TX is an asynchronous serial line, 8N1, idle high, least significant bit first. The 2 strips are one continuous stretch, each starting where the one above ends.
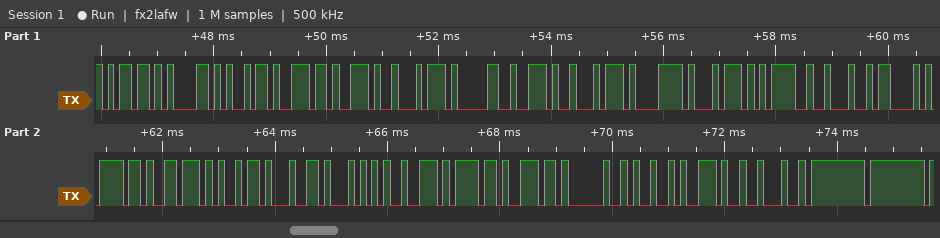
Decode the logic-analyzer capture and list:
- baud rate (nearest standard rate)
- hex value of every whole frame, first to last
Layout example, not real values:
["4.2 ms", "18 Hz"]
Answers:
["9600 baud", "6D 61 69 6E 2E 74 30 2E 74 78 74 3D 22 43 6F 76 69 64 54 72 6F 6E 20 49 2E 22 FF FF"]
